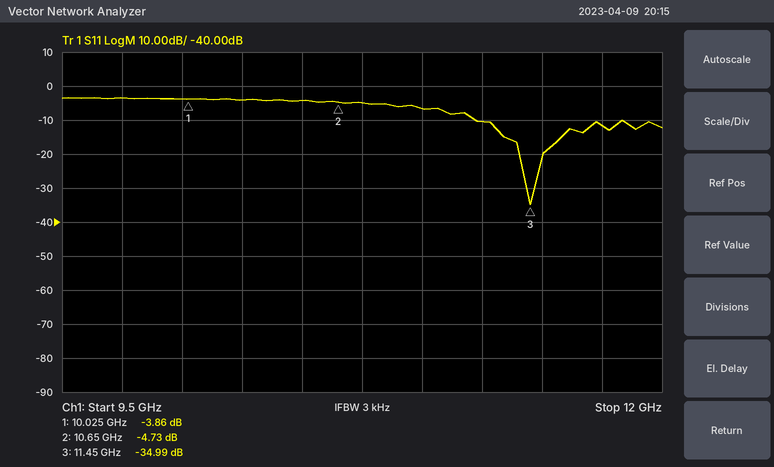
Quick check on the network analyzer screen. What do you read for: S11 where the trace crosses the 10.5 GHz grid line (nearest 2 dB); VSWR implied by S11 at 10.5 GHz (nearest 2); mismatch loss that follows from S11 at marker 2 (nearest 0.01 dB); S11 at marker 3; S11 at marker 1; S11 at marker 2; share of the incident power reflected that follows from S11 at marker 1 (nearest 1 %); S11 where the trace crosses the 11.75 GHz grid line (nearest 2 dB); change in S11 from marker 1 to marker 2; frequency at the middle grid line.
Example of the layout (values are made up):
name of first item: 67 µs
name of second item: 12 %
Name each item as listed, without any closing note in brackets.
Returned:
S11 where the trace crosses the 10.5 GHz grid line: -4 dB
VSWR implied by S11 at 10.5 GHz: 4
mismatch loss that follows from S11 at marker 2: 1.78 dB
S11 at marker 3: -34.99 dB
S11 at marker 1: -3.86 dB
S11 at marker 2: -4.73 dB
share of the incident power reflected that follows from S11 at marker 1: 41 %
S11 where the trace crosses the 11.75 GHz grid line: -12 dB
change in S11 from marker 1 to marker 2: -0.87 dB
frequency at the middle grid line: 10.75 GHz
